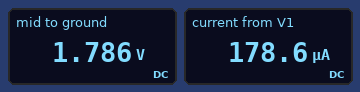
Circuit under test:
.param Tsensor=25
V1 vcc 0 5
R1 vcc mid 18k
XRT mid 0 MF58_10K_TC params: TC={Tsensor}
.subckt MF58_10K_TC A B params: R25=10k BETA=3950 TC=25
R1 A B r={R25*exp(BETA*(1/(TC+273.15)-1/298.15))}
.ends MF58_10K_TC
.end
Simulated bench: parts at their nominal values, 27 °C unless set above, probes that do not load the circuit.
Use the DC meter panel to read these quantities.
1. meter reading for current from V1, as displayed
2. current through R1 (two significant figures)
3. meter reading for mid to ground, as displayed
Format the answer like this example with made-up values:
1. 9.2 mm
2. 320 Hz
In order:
1. 178.6 µA
2. 180 µA
3. 1.786 V
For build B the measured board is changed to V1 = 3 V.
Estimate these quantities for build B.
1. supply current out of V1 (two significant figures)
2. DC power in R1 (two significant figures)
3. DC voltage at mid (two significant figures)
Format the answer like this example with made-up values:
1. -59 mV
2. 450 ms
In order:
1. 110 µA
2. 210 µW
3. 1.1 V
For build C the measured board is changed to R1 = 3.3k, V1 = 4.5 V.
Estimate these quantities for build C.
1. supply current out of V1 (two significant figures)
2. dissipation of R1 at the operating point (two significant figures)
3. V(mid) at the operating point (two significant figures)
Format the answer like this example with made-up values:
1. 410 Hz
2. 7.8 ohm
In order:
1. 340 µA
2. 380 µW
3. 3.4 V
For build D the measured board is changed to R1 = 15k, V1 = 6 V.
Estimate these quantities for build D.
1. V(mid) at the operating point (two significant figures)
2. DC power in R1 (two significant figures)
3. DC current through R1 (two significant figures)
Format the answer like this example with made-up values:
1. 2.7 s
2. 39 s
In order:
1. 2.4 V
2. 860 µW
3. 240 µA
